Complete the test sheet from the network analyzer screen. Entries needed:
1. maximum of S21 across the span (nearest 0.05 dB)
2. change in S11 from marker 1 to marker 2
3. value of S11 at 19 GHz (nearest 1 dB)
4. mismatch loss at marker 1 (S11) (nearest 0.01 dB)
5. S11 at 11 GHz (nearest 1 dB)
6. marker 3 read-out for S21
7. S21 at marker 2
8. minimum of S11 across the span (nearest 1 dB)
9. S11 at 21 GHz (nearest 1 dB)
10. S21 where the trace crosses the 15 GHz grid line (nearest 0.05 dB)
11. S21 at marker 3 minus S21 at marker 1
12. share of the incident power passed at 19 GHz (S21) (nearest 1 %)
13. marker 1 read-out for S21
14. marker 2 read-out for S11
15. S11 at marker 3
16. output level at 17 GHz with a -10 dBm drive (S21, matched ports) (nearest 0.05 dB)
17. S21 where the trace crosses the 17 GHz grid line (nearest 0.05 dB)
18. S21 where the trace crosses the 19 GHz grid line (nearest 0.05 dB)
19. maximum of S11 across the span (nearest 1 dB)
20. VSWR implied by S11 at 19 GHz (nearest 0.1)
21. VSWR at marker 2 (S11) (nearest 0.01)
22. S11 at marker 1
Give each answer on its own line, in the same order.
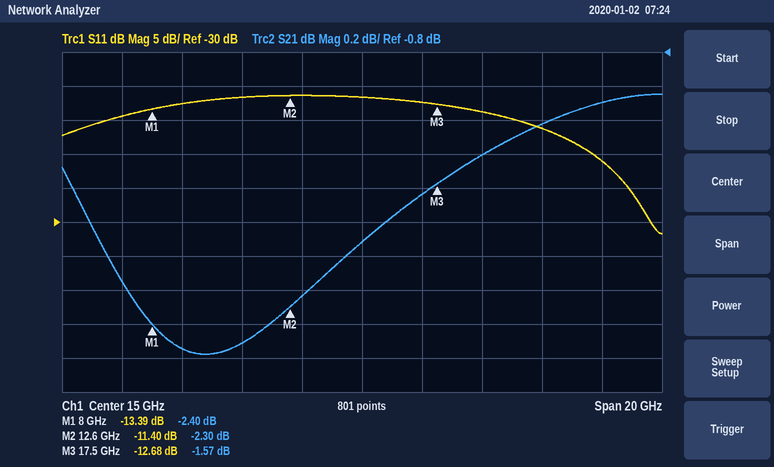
-1.05 dB
1.99 dB
-14 dB
0.20 dB
-12 dB
-1.57 dB
-2.30 dB
-32 dB
-16 dB
-1.90 dB
0.83 dB
72 %
-2.40 dB
-11.40 dB
-12.68 dB
-11.65 dBm
-1.65 dB
-1.40 dB
-11 dB
1.5
1.74
-13.39 dB
